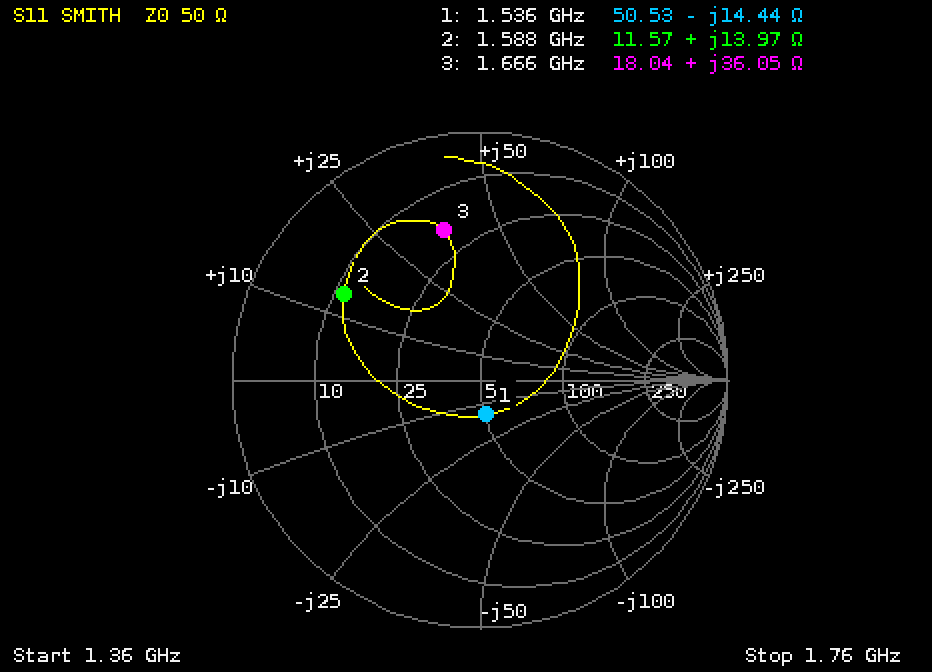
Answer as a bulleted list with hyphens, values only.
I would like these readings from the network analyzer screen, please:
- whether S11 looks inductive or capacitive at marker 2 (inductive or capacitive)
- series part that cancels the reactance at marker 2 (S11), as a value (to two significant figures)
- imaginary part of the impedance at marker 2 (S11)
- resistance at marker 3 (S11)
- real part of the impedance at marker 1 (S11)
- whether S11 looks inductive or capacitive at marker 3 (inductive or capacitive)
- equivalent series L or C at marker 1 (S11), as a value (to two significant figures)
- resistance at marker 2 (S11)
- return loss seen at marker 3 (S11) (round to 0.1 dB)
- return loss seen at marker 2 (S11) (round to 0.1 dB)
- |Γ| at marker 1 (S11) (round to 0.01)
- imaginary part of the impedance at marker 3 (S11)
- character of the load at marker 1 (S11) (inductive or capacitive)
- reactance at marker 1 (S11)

- inductive
- 7.2 pF
- +13.97 Ω
- 18.04 Ω
- 50.53 Ω
- inductive
- 7.2 pF
- 11.57 Ω
- 4.1 dB
- 3.8 dB
- 0.14
- +36.05 Ω
- capacitive
- -14.44 Ω
